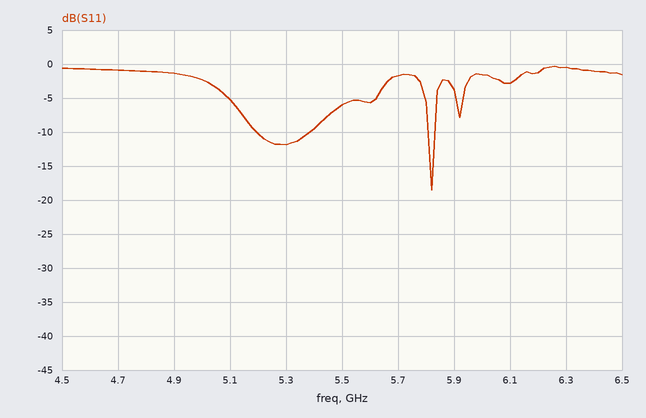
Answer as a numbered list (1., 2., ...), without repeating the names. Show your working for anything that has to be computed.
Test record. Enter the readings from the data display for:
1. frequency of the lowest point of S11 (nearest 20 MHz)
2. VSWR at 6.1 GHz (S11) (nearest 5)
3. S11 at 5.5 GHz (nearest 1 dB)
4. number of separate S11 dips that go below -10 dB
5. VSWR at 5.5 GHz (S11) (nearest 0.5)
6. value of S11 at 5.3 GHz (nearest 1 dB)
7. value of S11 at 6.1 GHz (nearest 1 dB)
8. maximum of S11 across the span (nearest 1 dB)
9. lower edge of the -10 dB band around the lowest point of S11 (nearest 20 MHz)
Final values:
1. 5.82 GHz
2. |Γ| = 10^(-3/20) = 0.7079; VSWR = (1 + 0.7079)/(1 − 0.7079) ≈ 5.85, so 5 to the nearest 5
3. -6 dB
4. 2
5. |Γ| = 10^(-6/20) = 0.5012; VSWR = (1 + 0.5012)/(1 − 0.5012) ≈ 3.0
6. -12 dB
7. -3 dB
8. 0 dB
9. 5.80 GHz
